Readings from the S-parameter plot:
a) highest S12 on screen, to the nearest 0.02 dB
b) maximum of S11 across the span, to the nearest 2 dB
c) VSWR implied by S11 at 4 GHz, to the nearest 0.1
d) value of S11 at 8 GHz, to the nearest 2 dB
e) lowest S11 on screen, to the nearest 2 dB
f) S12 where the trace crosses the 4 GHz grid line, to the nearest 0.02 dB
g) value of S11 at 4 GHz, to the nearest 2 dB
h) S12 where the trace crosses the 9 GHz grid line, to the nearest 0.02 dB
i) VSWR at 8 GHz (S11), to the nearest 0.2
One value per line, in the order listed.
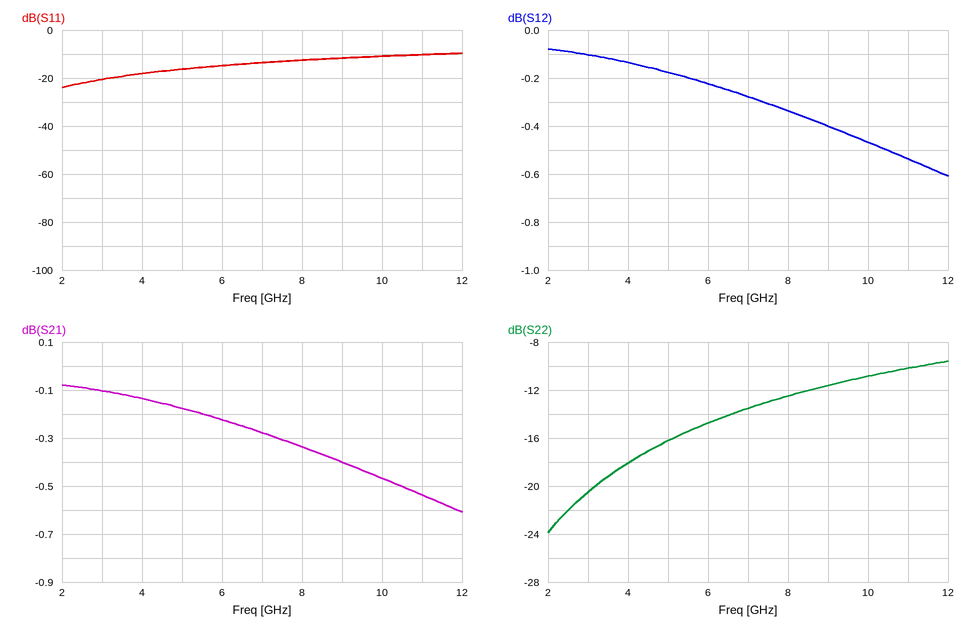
-0.08 dB
-10 dB
1.3
-12 dB
-24 dB
-0.14 dB
-18 dB
-0.40 dB
1.6
